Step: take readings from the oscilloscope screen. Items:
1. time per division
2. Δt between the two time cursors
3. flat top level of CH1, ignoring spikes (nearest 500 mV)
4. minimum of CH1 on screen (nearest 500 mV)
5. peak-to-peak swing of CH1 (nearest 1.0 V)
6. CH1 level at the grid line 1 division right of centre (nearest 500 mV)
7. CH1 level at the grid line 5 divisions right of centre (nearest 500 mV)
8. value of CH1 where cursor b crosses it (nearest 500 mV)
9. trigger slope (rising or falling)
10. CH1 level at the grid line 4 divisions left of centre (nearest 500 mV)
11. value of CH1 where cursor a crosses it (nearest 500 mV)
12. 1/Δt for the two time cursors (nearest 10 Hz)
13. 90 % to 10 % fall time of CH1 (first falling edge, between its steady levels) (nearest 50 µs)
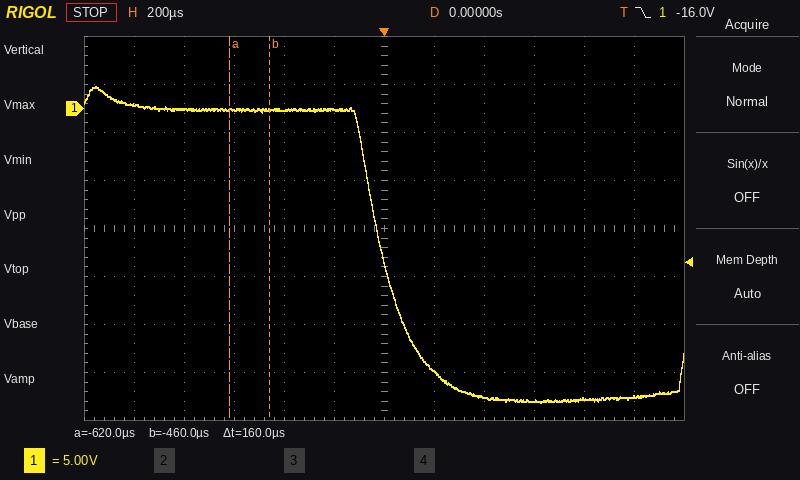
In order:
200 µs
160 µs
0.0 V
-30.5 V
33.0 V
-27.5 V
-30.0 V
0.0 V
falling
0.0 V
0.0 V
6.25 kHz
300 µs
